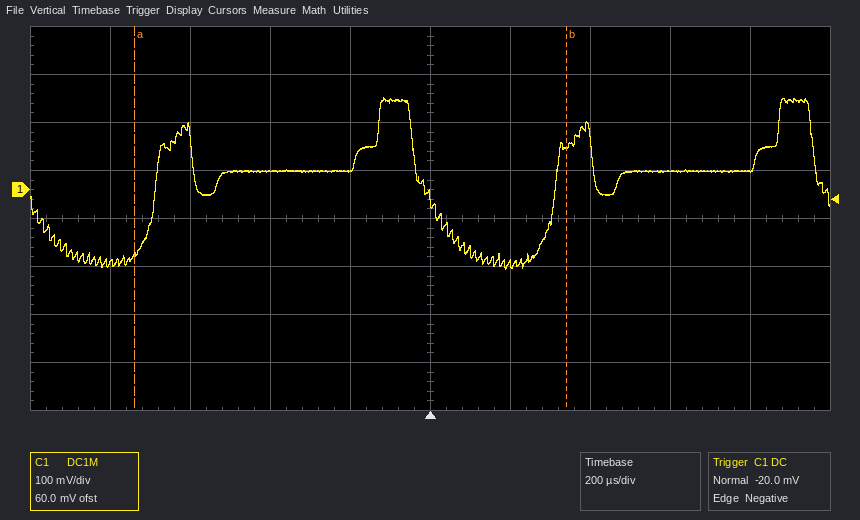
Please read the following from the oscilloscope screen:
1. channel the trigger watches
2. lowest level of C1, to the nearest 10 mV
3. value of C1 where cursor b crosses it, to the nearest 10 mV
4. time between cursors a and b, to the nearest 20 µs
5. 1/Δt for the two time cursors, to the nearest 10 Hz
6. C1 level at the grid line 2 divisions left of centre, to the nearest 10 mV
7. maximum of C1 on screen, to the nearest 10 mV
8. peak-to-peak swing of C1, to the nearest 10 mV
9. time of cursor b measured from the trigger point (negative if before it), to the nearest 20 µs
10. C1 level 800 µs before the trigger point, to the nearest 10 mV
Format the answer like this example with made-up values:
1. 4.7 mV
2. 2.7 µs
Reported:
1. C1
2. -170 mV
3. 90 mV
4. 1.08 ms
5. 930 Hz
6. 40 mV
7. 190 mV
8. 360 mV
9. +340 µs
10. -150 mV
